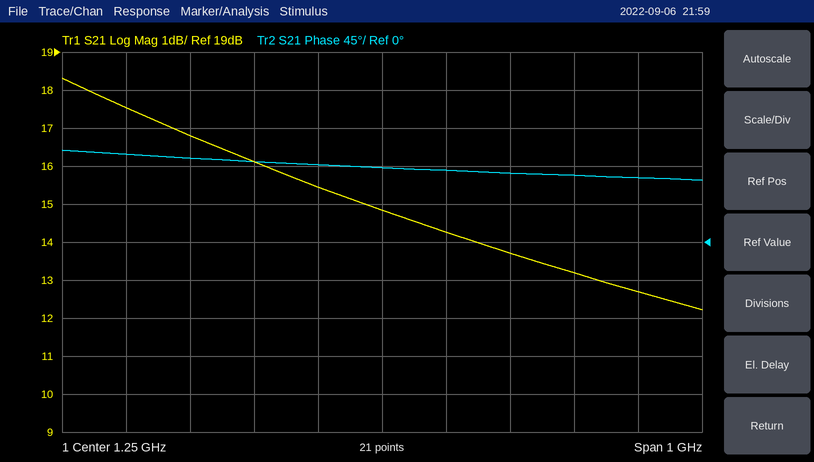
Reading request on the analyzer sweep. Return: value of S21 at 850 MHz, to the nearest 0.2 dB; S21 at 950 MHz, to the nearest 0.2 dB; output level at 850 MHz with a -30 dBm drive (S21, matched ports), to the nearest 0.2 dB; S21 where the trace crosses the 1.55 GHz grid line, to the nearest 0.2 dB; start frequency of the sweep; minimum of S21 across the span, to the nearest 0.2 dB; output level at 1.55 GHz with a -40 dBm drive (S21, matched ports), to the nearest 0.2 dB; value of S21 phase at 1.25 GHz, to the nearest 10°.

17.6 dB
16.8 dB
-12.4 dBm
13.2 dB
750 MHz
12.2 dB
-26.8 dBm
90°
